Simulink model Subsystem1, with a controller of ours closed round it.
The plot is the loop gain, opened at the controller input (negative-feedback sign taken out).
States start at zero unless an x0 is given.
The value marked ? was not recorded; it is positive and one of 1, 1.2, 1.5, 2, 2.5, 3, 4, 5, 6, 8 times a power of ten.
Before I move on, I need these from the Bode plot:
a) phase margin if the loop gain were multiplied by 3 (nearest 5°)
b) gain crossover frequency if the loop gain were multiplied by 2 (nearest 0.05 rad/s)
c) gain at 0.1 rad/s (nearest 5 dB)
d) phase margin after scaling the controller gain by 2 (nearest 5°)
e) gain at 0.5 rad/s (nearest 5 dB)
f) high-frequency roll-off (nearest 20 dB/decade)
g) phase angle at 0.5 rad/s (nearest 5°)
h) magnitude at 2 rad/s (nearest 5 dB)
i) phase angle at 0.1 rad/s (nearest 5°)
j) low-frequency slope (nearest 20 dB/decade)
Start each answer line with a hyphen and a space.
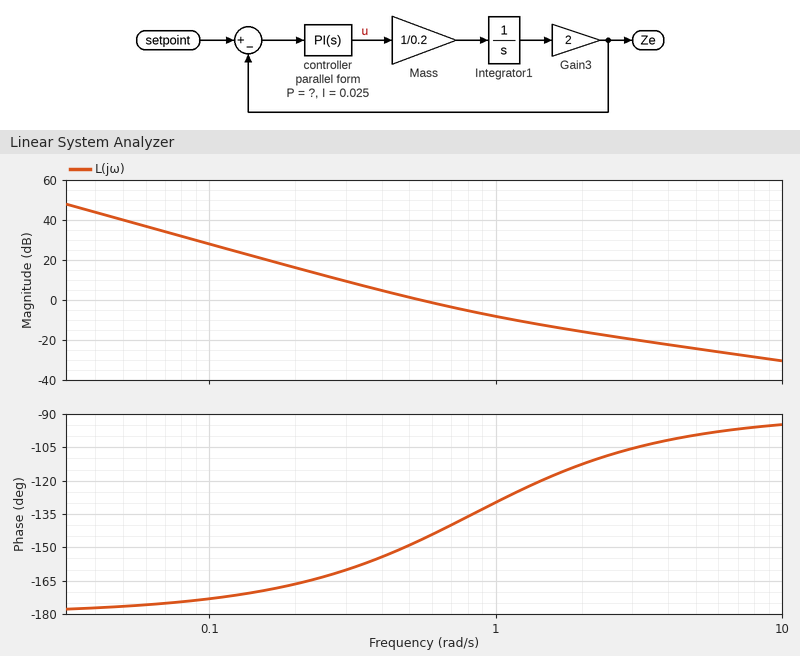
- 55°
- 0.85 rad/s
- 30 dB
- 45°
- 0 dB
- -20 dB/decade
- -150°
- -15 dB
- -175°
- -40 dB/decade
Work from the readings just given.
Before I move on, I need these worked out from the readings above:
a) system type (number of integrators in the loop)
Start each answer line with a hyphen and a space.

- 2
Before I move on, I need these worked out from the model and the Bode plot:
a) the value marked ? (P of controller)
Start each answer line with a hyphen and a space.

- 0.03
